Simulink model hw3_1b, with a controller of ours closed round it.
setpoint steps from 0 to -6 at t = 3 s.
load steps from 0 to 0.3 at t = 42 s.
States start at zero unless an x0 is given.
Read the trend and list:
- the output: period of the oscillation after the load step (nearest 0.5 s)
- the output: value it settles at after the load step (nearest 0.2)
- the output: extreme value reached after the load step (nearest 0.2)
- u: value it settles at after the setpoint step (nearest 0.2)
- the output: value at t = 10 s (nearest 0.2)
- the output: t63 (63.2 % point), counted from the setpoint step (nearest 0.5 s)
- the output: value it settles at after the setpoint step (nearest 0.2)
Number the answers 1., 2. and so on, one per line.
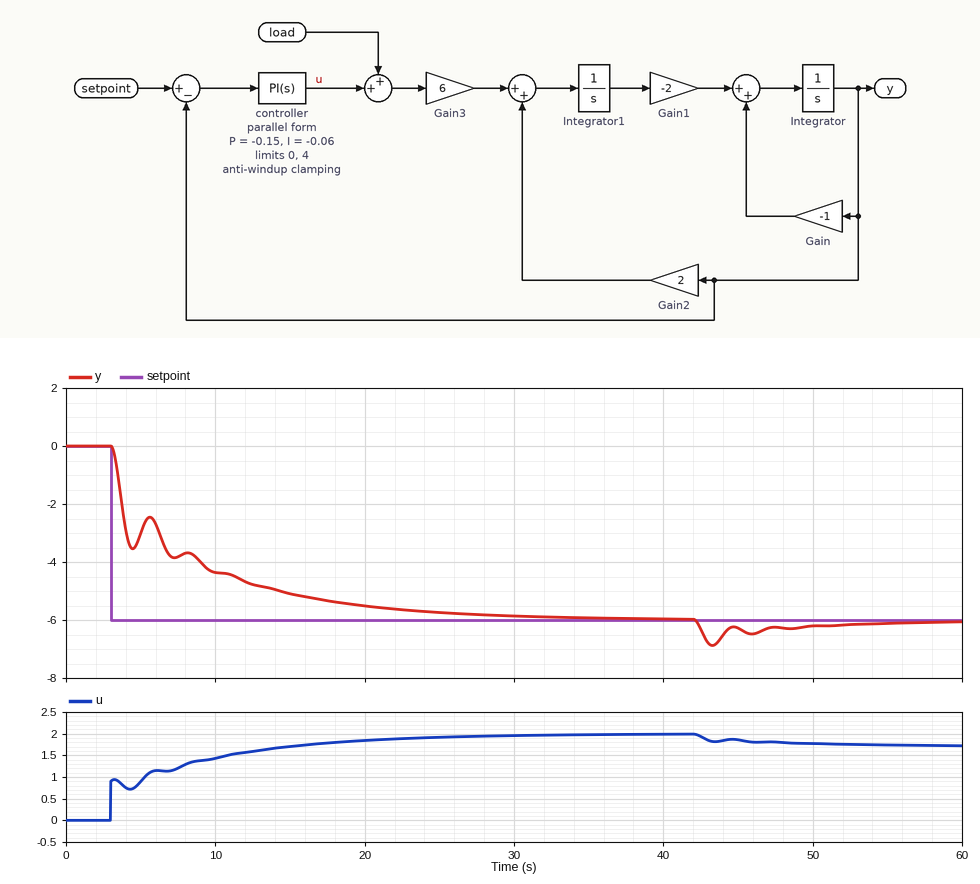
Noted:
1. 2.5 s
2. -6.0
3. -6.8
4. 2.0
5. -4.4
6. 4.0 s
7. -6.0
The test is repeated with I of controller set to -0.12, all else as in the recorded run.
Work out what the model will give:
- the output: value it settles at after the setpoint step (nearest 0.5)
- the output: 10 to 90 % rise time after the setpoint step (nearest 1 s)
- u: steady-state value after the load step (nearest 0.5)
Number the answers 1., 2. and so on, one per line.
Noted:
1. -6.0
2. 6 s
3. 1.5
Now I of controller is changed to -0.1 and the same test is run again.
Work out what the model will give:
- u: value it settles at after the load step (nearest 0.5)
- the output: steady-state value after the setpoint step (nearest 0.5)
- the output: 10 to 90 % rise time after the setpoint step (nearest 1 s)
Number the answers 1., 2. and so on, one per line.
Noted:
1. 1.5
2. -6.0
3. 9 s
